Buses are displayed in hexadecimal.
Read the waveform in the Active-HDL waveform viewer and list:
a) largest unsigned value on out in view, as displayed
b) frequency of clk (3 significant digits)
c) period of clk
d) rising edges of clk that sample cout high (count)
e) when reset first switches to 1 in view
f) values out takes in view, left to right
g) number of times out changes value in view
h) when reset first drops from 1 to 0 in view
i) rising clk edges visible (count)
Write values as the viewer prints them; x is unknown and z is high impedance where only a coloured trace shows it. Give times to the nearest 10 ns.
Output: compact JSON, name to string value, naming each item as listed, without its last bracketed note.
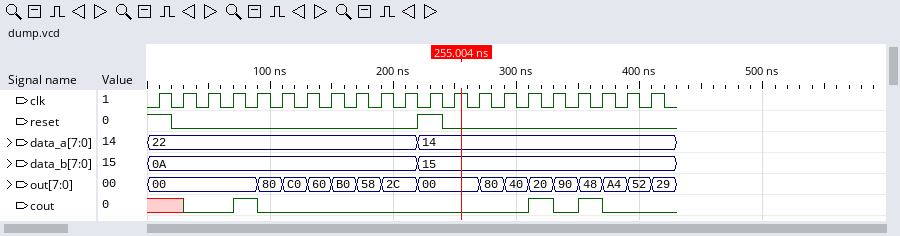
{"largest unsigned value on out in view, as displayed": "C0", "frequency of clk": "50.0 MHz", "period of clk": "20 ns", "rising edges of clk that sample cout high": "3", "when reset first switches to 1 in view": "220 ns", "values out takes in view, left to right": "00, 80, C0, 60, B0, 58, 2C, 00, 80, 40, 20, 90, 48, A4, 52, 29", "number of times out changes value in view": "15", "when reset first drops from 1 to 0 in view": "20 ns", "rising clk edges visible": "21"}
